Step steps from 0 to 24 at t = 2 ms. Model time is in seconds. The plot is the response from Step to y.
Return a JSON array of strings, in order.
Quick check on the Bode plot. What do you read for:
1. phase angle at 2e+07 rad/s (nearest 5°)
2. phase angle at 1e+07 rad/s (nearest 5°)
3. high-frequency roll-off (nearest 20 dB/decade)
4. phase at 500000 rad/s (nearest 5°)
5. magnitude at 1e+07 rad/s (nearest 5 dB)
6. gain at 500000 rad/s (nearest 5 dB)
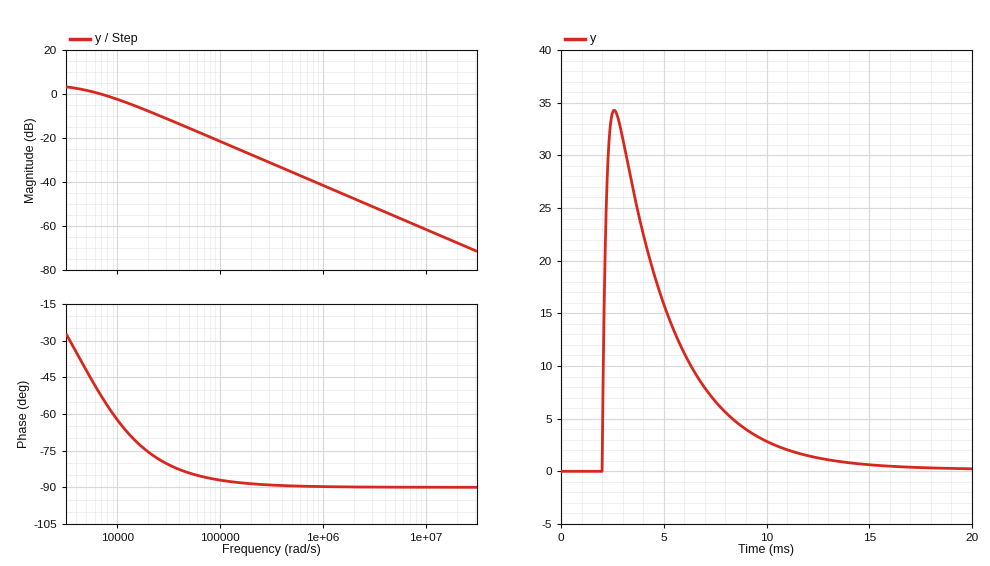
["-90°", "-90°", "-20 dB/decade", "-90°", "-60 dB", "-35 dB"]
